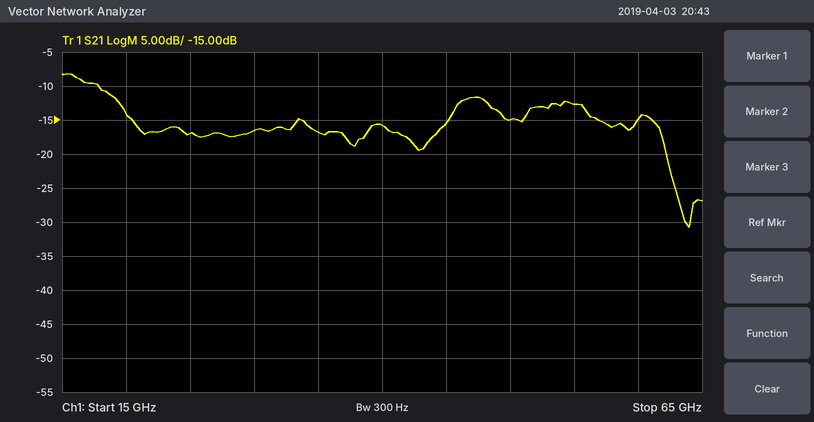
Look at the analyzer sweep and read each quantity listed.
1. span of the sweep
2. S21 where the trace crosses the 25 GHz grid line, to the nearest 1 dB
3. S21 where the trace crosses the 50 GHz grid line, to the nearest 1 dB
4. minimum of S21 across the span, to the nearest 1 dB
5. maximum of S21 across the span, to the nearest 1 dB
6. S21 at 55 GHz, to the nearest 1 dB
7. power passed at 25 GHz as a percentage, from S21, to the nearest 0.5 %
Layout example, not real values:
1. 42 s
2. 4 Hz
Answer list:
1. 50 GHz
2. -17 dB
3. -15 dB
4. -31 dB
5. -8 dB
6. -13 dB
7. 2.0 %
